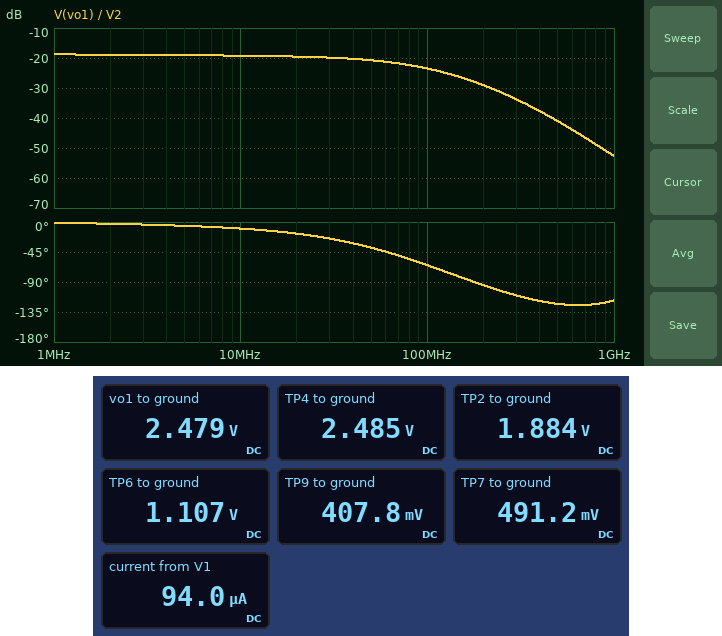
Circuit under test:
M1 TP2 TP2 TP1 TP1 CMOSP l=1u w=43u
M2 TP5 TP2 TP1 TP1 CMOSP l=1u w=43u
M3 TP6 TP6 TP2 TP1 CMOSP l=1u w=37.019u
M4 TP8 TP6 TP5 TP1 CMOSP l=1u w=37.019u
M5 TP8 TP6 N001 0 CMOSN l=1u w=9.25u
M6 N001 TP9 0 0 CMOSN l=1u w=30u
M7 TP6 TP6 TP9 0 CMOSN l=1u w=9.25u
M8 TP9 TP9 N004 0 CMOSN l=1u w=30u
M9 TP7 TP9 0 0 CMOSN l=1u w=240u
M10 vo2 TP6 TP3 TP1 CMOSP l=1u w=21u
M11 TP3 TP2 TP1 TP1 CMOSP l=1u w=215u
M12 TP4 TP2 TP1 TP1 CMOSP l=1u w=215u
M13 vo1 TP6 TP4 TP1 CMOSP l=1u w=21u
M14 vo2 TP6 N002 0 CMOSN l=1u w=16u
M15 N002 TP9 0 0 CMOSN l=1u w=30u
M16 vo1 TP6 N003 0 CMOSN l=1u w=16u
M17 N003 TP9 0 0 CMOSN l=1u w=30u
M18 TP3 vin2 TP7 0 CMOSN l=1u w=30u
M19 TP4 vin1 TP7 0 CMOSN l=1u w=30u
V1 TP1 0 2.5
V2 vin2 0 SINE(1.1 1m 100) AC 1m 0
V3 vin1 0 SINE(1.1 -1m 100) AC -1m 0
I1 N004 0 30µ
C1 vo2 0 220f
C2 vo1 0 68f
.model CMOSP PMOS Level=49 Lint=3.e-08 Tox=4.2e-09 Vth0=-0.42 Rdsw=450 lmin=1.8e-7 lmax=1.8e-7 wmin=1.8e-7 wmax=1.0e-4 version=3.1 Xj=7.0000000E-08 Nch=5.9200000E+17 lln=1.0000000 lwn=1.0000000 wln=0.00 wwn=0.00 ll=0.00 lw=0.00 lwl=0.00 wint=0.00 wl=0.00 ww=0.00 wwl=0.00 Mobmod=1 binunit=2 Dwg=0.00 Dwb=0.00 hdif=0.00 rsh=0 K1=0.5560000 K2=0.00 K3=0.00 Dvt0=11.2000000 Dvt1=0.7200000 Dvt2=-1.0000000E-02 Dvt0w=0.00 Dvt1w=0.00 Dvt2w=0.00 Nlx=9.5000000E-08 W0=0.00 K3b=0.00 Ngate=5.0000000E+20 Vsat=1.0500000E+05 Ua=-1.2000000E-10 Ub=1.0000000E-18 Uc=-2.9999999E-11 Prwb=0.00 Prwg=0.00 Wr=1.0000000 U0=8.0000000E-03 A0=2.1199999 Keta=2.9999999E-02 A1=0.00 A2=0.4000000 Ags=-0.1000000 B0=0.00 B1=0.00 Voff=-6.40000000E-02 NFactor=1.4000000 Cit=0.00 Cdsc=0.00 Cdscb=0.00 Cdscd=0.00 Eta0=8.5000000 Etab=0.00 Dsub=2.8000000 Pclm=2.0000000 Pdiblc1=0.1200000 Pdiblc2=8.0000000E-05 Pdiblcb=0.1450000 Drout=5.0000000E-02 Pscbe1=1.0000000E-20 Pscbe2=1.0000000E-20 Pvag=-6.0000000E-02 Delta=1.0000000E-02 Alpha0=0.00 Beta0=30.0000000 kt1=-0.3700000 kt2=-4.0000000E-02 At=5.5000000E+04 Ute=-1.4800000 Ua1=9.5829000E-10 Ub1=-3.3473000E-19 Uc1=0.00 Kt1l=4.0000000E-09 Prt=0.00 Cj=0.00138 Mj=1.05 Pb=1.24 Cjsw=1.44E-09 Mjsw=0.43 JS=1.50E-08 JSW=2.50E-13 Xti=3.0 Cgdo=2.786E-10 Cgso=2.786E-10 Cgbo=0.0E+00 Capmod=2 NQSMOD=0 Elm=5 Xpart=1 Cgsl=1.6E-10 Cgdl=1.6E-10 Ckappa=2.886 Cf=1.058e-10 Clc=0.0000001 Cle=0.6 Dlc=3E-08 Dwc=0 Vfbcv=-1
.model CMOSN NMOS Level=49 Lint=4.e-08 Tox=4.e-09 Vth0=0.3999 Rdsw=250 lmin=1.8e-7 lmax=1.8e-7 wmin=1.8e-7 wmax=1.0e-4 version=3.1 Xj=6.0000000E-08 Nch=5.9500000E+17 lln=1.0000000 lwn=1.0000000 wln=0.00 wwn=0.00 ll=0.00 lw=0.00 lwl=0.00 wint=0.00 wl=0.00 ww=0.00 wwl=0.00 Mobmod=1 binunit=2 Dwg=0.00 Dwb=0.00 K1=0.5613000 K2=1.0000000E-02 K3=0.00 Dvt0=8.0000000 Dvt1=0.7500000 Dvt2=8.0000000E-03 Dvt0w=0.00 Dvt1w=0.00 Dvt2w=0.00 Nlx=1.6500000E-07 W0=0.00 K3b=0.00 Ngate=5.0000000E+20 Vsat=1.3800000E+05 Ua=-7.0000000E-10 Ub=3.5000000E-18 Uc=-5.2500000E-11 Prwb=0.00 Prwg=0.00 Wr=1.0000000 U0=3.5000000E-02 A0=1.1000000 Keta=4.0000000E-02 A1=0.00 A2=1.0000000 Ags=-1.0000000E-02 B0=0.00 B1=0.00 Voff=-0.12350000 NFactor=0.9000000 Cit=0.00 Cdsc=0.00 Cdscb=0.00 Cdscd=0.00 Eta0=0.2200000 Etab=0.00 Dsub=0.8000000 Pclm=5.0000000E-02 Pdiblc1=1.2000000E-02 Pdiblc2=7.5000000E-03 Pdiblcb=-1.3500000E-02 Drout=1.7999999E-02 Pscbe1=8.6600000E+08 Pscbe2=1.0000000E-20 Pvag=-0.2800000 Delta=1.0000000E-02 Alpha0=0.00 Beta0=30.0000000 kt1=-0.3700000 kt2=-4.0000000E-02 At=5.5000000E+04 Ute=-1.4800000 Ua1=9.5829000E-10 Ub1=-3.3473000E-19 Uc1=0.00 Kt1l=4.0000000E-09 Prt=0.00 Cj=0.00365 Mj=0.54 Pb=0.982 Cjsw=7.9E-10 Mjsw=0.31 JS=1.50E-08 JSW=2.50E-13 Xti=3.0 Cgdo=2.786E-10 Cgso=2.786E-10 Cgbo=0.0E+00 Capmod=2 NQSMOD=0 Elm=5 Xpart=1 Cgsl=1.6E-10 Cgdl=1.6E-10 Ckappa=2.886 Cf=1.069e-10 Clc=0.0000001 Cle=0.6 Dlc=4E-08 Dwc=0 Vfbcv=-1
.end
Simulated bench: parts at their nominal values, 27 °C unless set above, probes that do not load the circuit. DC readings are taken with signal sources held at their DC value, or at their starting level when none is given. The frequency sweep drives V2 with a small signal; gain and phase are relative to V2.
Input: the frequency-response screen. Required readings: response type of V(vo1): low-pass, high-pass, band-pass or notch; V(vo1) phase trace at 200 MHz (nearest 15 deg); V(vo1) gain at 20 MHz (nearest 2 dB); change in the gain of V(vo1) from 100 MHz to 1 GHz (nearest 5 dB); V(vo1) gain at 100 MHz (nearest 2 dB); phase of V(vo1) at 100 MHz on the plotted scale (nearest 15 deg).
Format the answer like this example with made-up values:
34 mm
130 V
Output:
low-pass
-90 deg
-20 dB
-30 dB
-24 dB
-60 deg
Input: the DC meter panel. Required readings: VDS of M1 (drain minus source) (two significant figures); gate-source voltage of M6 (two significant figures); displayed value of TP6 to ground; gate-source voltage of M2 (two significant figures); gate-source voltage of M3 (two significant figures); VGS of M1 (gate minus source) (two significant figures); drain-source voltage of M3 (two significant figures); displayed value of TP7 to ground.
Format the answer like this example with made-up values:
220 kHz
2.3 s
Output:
-620 mV
410 mV
1.107 V
-620 mV
-780 mV
-620 mV
-780 mV
491.2 mV
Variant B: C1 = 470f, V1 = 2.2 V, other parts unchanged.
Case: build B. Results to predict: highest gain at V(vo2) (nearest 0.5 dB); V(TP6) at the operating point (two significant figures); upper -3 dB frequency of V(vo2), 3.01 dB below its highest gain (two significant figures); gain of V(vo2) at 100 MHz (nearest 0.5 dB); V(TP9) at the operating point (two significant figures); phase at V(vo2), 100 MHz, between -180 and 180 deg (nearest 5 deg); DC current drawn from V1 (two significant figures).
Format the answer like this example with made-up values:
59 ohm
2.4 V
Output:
-49.5 dB
810 mV
500 MHz
-50.5 dB
170 mV
35 deg
30 µA
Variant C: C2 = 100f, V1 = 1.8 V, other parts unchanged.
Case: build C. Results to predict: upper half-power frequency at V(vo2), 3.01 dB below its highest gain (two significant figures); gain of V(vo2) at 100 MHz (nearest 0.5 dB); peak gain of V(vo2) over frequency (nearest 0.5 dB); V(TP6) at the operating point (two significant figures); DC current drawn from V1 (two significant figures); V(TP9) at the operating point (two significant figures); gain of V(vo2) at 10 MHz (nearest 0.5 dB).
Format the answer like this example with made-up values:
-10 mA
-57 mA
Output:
670 MHz
-49.5 dB
-48.0 dB
420 mV
28 µA
-120 mV
-66.0 dB
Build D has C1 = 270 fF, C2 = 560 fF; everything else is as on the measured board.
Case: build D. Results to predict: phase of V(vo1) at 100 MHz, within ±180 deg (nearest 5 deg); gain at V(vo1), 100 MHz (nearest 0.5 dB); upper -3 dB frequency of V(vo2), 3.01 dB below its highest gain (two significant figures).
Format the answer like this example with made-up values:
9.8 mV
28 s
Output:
-80 deg
-25.0 dB
97 MHz
